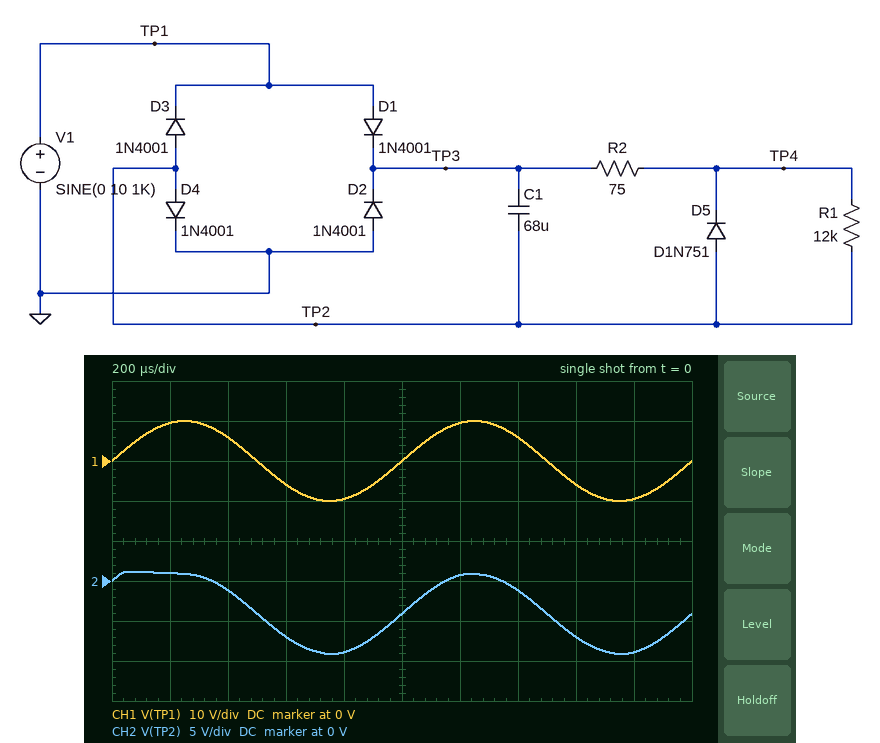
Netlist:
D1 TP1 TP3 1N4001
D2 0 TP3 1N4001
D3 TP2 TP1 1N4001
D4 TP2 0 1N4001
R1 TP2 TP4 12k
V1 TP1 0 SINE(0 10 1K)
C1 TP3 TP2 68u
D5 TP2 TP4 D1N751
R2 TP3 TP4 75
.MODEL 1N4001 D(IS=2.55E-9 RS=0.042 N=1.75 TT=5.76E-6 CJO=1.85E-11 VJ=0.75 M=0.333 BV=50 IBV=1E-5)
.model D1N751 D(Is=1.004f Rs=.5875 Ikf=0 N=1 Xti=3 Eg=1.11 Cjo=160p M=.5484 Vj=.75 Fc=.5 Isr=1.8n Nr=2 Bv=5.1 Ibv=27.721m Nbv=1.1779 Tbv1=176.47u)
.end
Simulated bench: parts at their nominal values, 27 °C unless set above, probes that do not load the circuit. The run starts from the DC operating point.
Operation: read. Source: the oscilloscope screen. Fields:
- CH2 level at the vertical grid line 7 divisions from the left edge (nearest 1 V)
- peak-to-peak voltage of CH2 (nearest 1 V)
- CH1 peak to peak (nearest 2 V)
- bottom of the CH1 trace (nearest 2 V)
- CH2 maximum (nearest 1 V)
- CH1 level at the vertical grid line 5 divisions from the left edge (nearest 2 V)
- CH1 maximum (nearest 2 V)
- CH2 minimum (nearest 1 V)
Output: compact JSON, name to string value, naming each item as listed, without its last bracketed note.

{"CH2 level at the vertical grid line 7 divisions from the left edge": "-1 V", "peak-to-peak voltage of CH2": "10 V", "CH1 peak to peak": "20 V", "bottom of the CH1 trace": "-10 V", "CH2 maximum": "1 V", "CH1 level at the vertical grid line 5 divisions from the left edge": "0 V", "CH1 maximum": "10 V", "CH2 minimum": "-9 V"}
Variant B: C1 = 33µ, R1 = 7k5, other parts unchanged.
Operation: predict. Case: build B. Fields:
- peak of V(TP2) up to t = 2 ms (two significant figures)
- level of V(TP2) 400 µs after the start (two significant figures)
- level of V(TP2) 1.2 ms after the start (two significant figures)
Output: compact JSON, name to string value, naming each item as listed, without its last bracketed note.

{"peak of V(TP2) up to t = 2 ms": "1.0 V", "level of V(TP2) 400 µs after the start": "-1.2 V", "level of V(TP2) 1.2 ms after the start": "810 mV"}
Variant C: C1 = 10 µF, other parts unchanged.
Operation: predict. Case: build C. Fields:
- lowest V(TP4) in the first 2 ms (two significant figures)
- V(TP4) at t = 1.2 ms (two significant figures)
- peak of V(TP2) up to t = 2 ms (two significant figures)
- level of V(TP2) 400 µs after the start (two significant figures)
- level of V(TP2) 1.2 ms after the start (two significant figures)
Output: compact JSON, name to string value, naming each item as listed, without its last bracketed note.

{"lowest V(TP4) in the first 2 ms": "-4.1 V", "V(TP4) at t = 1.2 ms": "6.0 V", "peak of V(TP2) up to t = 2 ms": "900 mV", "level of V(TP2) 400 µs after the start": "-1.0 V", "level of V(TP2) 1.2 ms after the start": "840 mV"}
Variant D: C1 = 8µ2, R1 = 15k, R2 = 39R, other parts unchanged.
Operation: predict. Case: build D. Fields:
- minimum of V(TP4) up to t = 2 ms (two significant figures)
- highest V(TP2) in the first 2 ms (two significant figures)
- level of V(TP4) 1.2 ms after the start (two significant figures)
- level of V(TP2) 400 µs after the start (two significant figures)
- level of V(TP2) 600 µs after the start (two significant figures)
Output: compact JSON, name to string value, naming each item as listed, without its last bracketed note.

{"minimum of V(TP4) up to t = 2 ms": "-4.0 V", "highest V(TP2) in the first 2 ms": "880 mV", "level of V(TP4) 1.2 ms after the start": "6.0 V", "level of V(TP2) 400 µs after the start": "-740 mV", "level of V(TP2) 600 µs after the start": "-6.1 V"}
